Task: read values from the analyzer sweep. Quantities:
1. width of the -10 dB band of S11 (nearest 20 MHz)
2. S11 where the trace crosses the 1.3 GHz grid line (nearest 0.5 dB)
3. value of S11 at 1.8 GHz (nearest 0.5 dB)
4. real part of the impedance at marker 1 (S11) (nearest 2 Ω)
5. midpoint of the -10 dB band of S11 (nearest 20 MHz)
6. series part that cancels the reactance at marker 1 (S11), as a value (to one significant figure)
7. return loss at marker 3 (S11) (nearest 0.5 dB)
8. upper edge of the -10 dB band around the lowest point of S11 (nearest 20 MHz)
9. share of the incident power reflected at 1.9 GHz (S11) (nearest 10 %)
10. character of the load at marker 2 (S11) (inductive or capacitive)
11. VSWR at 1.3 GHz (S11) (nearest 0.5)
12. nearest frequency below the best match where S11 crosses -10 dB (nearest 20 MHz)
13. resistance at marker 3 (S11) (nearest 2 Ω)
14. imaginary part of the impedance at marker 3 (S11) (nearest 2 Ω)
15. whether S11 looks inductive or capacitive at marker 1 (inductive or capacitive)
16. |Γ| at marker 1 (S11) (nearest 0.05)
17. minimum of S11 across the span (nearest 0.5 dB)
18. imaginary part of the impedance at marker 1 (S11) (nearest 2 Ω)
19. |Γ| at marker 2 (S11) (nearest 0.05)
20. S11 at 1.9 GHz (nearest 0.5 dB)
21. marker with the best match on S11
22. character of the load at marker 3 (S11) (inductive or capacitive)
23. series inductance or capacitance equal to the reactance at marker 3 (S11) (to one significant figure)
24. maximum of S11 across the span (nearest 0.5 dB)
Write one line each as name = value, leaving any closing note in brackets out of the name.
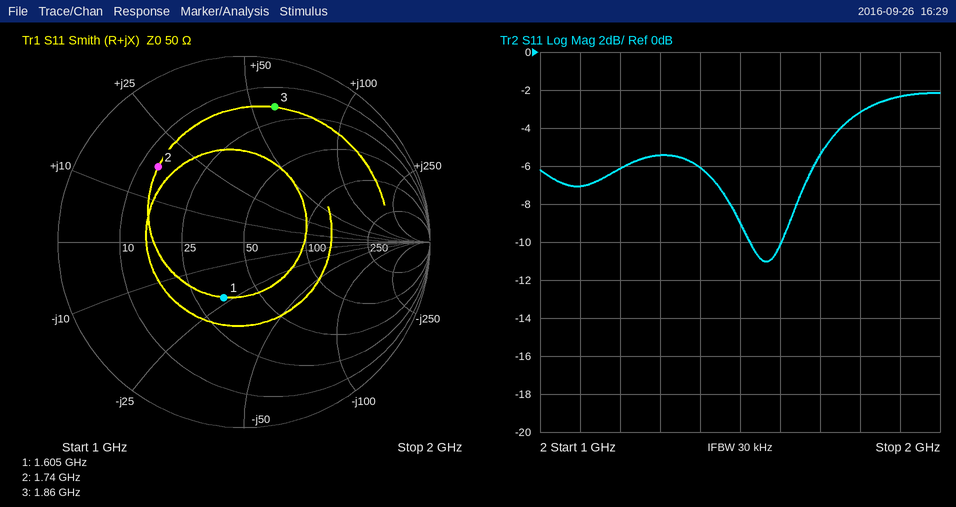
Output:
width of the -10 dB band of S11 = 80 MHz
S11 where the trace crosses the 1.3 GHz grid line = -5.5 dB
value of S11 at 1.8 GHz = -3.0 dB
real part of the impedance at marker 1 (S11) = 34 Ω
midpoint of the -10 dB band of S11 = 1.56 GHz
series part that cancels the reactance at marker 1 (S11), as a value = 2 nH
return loss at marker 3 (S11) = 2.5 dB
upper edge of the -10 dB band around the lowest point of S11 = 1.60 GHz
share of the incident power reflected at 1.9 GHz (S11) = 60 %
character of the load at marker 2 (S11) = inductive
VSWR at 1.3 GHz (S11) = 3.5
nearest frequency below the best match where S11 crosses -10 dB = 1.52 GHz
resistance at marker 3 (S11) = 18 Ω
imaginary part of the impedance at marker 3 (S11) = +60 Ω
whether S11 looks inductive or capacitive at marker 1 = capacitive
|Γ| at marker 1 (S11) = 0.30
minimum of S11 across the span = -11.0 dB
imaginary part of the impedance at marker 1 (S11) = -22 Ω
|Γ| at marker 2 (S11) = 0.60
S11 at 1.9 GHz = -2.5 dB
marker with the best match on S11 = marker 1
character of the load at marker 3 (S11) = inductive
series inductance or capacitance equal to the reactance at marker 3 (S11) = 5 nH
maximum of S11 across the span = -2.0 dB
